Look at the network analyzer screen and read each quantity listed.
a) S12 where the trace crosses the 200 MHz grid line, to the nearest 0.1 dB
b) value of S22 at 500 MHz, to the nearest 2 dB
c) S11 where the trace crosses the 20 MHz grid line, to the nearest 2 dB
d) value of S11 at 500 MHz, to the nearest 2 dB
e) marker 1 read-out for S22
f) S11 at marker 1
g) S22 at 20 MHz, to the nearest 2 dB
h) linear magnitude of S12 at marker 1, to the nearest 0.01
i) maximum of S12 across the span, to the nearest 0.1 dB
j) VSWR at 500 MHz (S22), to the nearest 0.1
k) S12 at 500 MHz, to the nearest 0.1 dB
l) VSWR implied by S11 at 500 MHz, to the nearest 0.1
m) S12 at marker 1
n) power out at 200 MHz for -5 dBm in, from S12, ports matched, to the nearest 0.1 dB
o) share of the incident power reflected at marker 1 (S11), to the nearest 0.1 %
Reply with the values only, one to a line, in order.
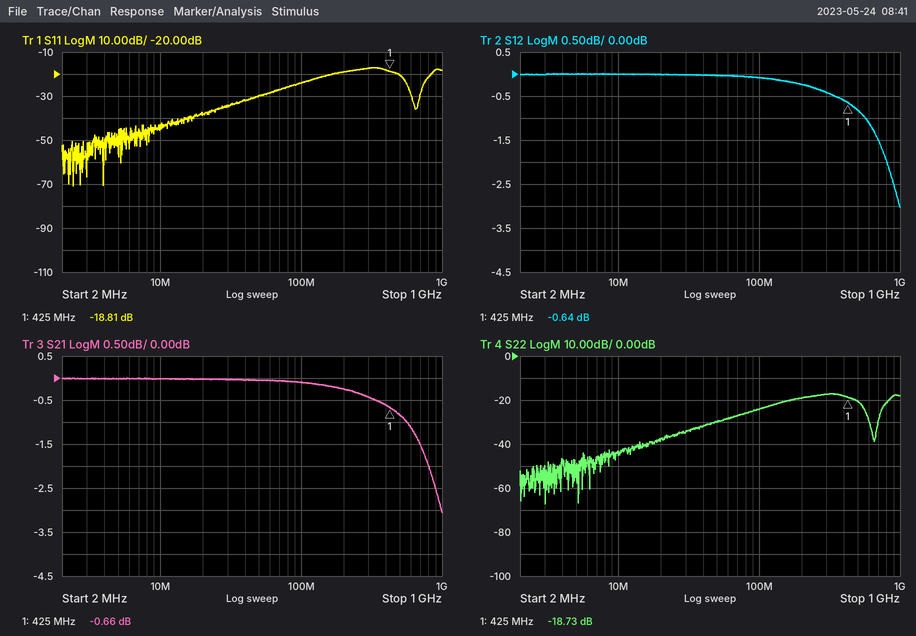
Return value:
-0.2 dB
-20 dB
-38 dB
-20 dB
-18.73 dB
-18.81 dB
-38 dB
0.93
0.0 dB
1.2
-0.8 dB
1.2
-0.64 dB
-5.2 dBm
1.3 %
